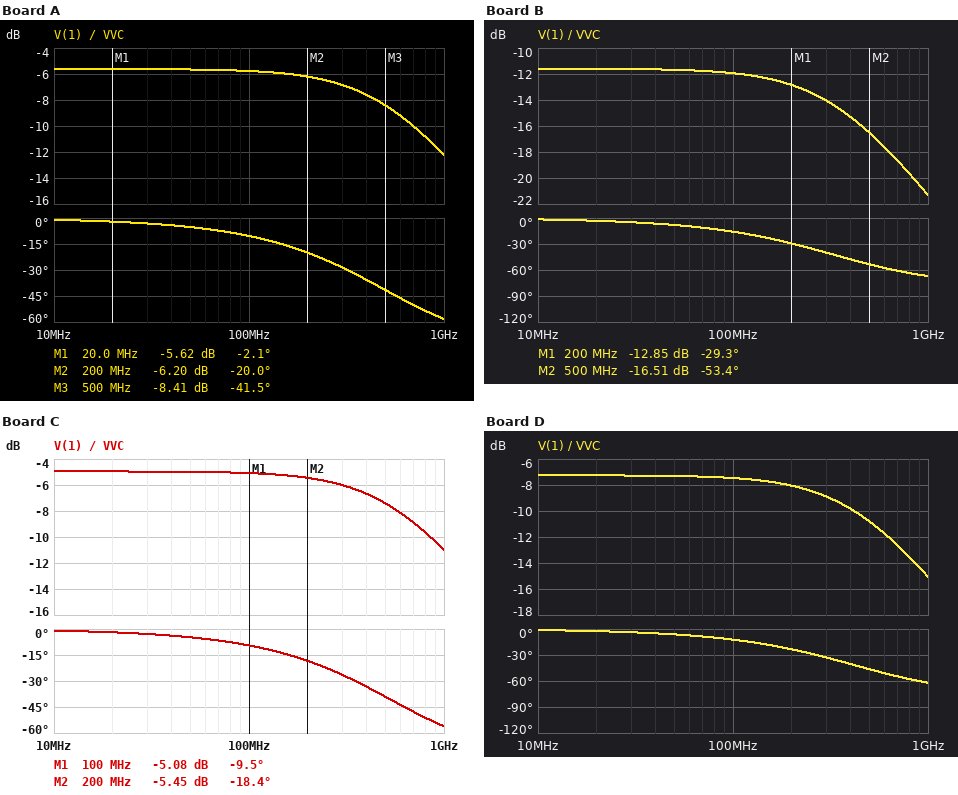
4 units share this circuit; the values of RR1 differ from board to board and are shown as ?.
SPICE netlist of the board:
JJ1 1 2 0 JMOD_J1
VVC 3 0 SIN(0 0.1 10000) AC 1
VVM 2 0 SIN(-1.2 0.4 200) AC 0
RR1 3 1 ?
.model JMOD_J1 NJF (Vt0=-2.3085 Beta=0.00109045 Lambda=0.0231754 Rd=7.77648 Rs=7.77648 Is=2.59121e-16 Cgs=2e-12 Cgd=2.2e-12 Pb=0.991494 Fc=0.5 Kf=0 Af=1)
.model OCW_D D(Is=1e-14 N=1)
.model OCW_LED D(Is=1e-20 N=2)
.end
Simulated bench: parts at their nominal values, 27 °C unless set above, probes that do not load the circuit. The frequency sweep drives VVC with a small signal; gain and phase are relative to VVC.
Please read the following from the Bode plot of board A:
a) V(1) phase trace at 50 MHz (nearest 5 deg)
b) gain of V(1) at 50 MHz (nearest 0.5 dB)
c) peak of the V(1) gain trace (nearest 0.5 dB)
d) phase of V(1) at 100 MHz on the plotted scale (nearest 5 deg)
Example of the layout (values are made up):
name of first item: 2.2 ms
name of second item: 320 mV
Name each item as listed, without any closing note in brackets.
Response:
V(1) phase trace at 50 MHz: -5 deg
gain of V(1) at 50 MHz: -5.5 dB
peak of the V(1) gain trace: -5.5 dB
phase of V(1) at 100 MHz on the plotted scale: -10 deg
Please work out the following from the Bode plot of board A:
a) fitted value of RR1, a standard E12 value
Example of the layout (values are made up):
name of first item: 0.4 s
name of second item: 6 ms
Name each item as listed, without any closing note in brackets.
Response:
fitted value of RR1, a standard E12 value: 390 Ω
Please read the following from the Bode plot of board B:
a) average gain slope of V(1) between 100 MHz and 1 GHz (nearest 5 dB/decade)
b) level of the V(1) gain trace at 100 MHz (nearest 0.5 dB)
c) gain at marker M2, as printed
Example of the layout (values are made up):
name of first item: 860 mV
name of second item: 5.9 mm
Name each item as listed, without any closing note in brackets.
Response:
average gain slope of V(1) between 100 MHz and 1 GHz: -10 dB/decade
level of the V(1) gain trace at 100 MHz: -12.0 dB
gain at marker M2, as printed: -16.51 dB
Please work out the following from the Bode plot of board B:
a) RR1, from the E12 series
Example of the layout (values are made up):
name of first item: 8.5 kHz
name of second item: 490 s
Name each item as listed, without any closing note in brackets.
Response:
RR1, from the E12 series: 1.2 kΩ
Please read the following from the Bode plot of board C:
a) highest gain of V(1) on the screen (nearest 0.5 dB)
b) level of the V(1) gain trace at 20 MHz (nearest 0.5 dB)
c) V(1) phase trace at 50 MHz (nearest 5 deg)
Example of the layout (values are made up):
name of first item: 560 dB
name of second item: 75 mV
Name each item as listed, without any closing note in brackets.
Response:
highest gain of V(1) on the screen: -5.0 dB
level of the V(1) gain trace at 20 MHz: -5.0 dB
V(1) phase trace at 50 MHz: -5 deg
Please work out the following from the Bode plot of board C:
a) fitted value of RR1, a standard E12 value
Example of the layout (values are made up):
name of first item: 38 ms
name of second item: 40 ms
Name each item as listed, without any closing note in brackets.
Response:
fitted value of RR1, a standard E12 value: 330 Ω
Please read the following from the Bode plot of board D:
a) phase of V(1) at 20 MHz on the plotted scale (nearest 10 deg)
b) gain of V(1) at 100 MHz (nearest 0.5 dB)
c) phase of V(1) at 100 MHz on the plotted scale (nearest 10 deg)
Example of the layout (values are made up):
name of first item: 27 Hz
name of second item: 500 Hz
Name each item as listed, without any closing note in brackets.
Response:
phase of V(1) at 20 MHz on the plotted scale: 0 deg
gain of V(1) at 100 MHz: -7.5 dB
phase of V(1) at 100 MHz on the plotted scale: -10 deg
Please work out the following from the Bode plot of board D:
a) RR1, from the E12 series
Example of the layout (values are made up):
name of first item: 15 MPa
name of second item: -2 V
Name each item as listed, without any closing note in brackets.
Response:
RR1, from the E12 series: 560 Ω
